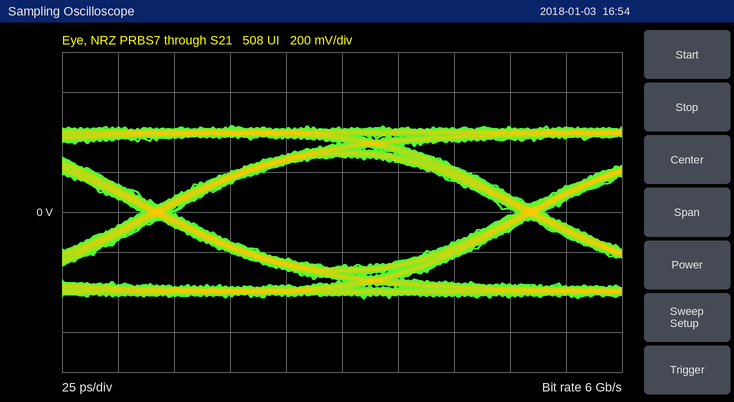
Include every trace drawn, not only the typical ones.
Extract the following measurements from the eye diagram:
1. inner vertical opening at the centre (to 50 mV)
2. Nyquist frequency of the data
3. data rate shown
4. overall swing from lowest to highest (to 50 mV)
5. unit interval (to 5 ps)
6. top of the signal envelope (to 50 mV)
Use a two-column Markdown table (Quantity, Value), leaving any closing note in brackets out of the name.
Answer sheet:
| Quantity | Value |
|---|---|
| inner vertical opening at the centre | 550 mV |
| Nyquist frequency of the data | 3 GHz |
| data rate shown | 6 Gb/s |
| overall swing from lowest to highest | 850 mV |
| unit interval | 165 ps |
| top of the signal envelope | 450 mV |
